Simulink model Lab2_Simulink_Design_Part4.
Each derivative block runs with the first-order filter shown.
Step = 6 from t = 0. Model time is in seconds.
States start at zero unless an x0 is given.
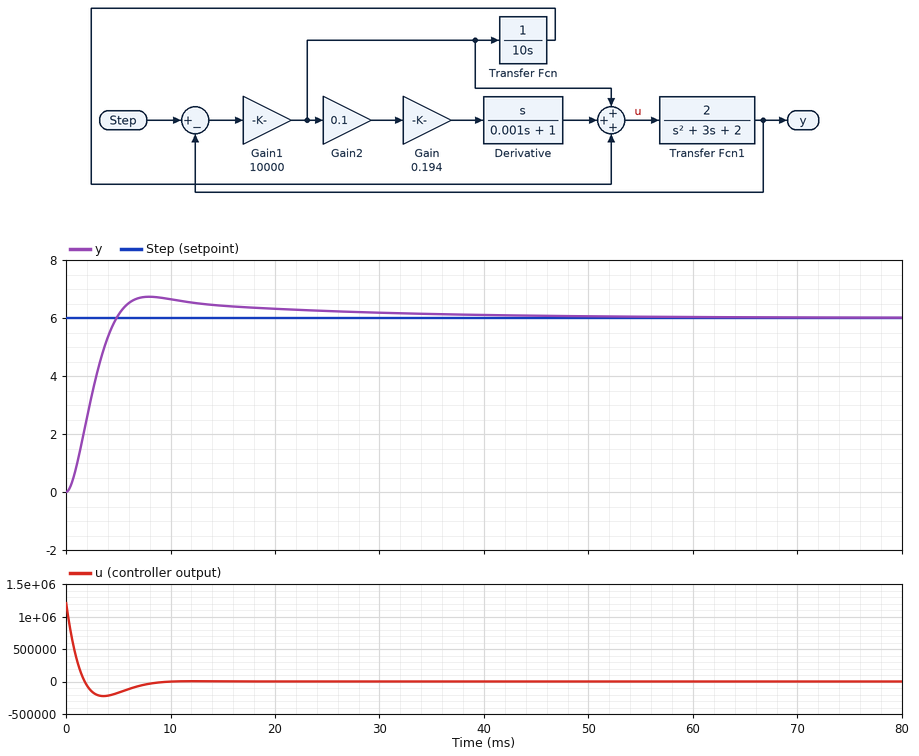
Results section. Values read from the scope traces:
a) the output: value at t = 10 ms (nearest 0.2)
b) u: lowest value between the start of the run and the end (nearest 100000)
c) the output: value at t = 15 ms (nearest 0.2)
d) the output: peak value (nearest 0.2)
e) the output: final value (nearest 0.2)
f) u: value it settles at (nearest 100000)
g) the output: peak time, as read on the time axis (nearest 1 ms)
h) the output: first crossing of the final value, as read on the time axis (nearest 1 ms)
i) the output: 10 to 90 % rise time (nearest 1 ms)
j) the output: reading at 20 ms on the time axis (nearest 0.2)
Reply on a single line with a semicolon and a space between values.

6.6; -200000; 6.4; 6.8; 6.0; 0; 8 ms; 5 ms; 3 ms; 6.4
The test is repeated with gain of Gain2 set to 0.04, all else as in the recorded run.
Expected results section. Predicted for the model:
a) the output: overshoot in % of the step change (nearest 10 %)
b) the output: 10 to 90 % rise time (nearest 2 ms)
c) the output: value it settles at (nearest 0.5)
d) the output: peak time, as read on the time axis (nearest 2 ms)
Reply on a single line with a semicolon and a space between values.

30 %; 6 ms; 6.0; 16 ms
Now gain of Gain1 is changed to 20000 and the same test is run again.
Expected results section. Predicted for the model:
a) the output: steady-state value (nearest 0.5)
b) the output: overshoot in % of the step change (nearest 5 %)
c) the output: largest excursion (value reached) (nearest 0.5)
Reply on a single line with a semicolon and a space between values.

6.0; 20 %; 7.0
